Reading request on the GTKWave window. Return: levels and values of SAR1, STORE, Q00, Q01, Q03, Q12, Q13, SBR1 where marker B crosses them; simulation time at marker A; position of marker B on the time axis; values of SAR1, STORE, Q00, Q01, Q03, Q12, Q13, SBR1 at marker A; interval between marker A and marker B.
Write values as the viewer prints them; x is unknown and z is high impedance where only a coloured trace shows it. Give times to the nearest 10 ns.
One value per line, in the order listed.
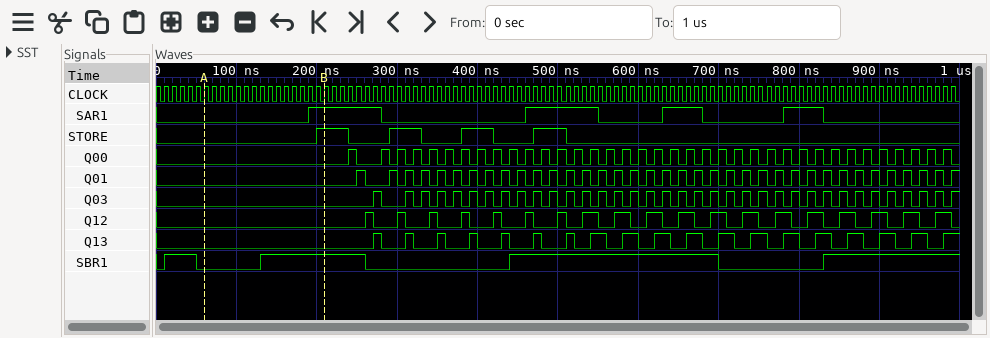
SAR1=1, STORE=1, Q00=0, Q01=0, Q03=0, Q12=0, Q13=0, SBR1=1
60 ns
210 ns
SAR1=0, STORE=0, Q00=0, Q01=0, Q03=0, Q12=0, Q13=0, SBR1=0
150 ns
